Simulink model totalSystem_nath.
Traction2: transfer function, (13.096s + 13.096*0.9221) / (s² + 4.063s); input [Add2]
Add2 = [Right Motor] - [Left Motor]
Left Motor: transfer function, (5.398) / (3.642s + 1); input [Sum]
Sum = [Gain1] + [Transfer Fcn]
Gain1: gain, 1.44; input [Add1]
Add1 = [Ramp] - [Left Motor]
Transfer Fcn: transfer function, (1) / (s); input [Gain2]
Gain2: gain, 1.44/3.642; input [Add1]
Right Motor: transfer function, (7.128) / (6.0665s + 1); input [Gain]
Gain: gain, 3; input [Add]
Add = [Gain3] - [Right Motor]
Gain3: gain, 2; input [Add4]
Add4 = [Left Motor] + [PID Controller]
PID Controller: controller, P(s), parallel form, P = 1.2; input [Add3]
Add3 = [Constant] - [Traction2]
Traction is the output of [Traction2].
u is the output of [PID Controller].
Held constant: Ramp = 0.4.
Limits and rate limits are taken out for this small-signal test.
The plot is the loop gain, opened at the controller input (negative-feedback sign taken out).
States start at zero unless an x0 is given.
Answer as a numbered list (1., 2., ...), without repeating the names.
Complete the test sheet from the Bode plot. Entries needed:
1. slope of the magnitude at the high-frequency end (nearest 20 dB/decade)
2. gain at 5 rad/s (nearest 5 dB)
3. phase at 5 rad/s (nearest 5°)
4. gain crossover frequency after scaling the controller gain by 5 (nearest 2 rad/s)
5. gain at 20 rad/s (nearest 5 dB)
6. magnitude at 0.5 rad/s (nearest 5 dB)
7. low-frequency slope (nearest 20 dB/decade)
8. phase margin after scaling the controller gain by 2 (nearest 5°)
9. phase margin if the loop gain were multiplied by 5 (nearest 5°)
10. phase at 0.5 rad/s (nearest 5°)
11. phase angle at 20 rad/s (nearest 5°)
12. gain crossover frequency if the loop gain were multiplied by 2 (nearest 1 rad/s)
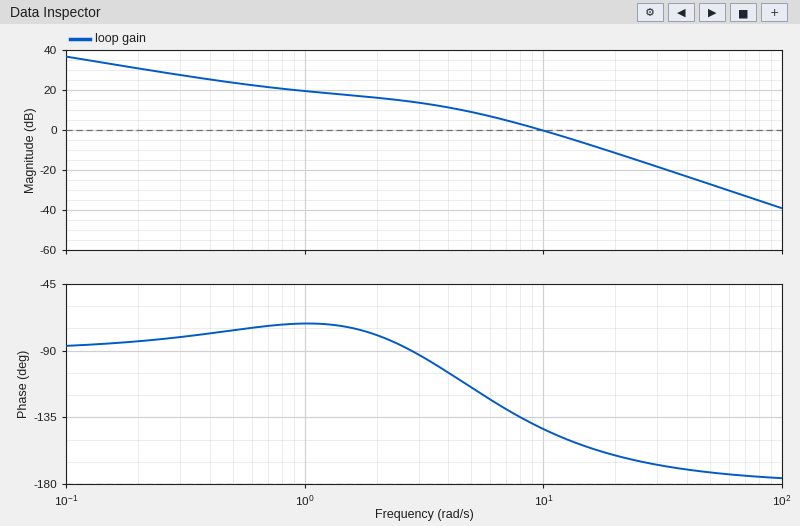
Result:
1. -40 dB/decade
2. 10 dB
3. -115°
4. 24 rad/s
5. -10 dB
6. 25 dB
7. -20 dB/decade
8. 25°
9. 15°
10. -75°
11. -160°
12. 14 rad/s
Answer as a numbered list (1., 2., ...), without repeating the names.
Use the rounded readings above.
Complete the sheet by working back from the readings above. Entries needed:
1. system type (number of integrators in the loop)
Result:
1. 1
